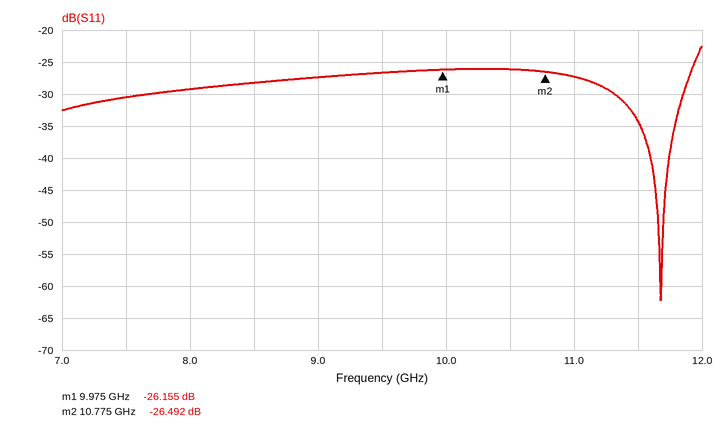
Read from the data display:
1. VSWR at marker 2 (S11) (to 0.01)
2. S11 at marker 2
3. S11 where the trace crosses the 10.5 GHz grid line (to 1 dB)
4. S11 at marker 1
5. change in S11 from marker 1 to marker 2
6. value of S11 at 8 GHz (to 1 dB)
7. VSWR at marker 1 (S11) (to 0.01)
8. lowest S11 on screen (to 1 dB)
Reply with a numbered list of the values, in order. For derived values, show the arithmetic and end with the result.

1. (1 + 0.0474)/(1 − 0.0474) ≈ 1.10
2. -26.492 dB
3. -26 dB
4. -26.155 dB
5. -26.492 − (-26.155) = -0.337 dB
6. -29 dB
7. (1 + 0.0492)/(1 − 0.0492) ≈ 1.10
8. -62 dB
